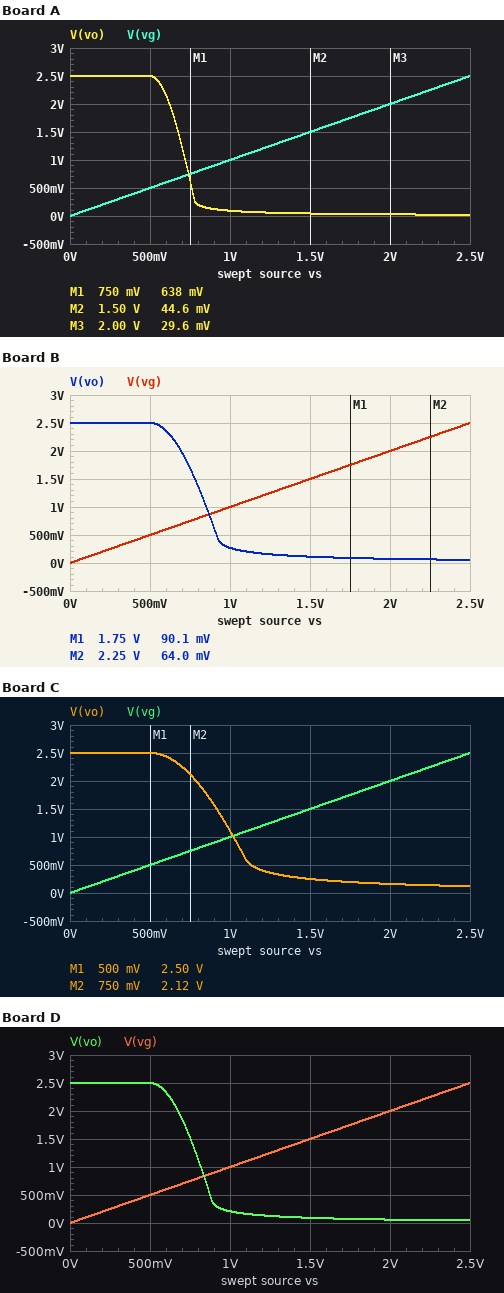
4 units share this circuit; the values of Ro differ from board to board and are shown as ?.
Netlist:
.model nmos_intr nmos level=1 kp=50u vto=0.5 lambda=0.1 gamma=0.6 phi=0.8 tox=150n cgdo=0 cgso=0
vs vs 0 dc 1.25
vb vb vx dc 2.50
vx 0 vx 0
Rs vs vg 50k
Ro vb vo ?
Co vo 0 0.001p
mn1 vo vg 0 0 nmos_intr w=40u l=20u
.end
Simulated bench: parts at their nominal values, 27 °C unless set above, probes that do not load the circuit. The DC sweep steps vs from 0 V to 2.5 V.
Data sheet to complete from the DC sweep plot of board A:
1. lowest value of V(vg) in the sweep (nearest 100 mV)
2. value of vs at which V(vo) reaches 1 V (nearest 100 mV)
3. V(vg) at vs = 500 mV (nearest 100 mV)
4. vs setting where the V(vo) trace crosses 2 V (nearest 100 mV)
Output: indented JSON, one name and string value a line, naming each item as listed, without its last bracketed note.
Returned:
{
  "lowest value of V(vg) in the sweep": "0 V",
  "value of vs at which V(vo) reaches 1 V": "700 mV",
  "V(vg) at vs = 500 mV": "500 mV",
  "vs setting where the V(vo) trace crosses 2 V": "600 mV"
}
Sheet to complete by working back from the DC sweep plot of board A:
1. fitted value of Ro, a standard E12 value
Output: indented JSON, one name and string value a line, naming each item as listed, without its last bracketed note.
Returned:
{
  "fitted value of Ro, a standard E12 value": "560 kΩ"
}
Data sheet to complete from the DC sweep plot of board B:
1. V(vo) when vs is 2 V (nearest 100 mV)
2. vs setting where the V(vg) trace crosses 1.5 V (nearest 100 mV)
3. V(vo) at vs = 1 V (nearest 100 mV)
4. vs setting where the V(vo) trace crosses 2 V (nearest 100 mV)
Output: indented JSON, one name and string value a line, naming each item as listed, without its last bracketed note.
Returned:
{
  "V(vo) when vs is 2 V": "100 mV",
  "vs setting where the V(vg) trace crosses 1.5 V": "1.5 V",
  "V(vo) at vs = 1 V": "300 mV",
  "vs setting where the V(vo) trace crosses 2 V": "700 mV"
}
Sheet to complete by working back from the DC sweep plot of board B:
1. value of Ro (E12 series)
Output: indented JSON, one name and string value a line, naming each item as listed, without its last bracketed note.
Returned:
{
  "value of Ro": "220 kΩ"
}
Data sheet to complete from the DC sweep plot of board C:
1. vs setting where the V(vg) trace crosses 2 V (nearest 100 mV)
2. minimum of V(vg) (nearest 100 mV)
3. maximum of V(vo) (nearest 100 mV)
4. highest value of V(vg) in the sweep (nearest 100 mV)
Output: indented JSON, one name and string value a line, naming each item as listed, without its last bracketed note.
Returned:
{
  "vs setting where the V(vg) trace crosses 2 V": "2.0 V",
  "minimum of V(vg)": "0 V",
  "maximum of V(vo)": "2.5 V",
  "highest value of V(vg) in the sweep": "2.5 V"
}
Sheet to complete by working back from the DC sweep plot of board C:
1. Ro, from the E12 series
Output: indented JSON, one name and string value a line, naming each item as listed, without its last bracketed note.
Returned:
{
  "Ro, from the E12 series": "100 kΩ"
}
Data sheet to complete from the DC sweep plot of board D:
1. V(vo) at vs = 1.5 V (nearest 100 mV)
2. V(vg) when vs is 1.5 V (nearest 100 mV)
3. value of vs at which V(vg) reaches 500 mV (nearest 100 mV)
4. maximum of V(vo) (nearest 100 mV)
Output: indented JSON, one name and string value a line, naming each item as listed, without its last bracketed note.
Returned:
{
  "V(vo) at vs = 1.5 V": "100 mV",
  "V(vg) when vs is 1.5 V": "1.5 V",
  "value of vs at which V(vg) reaches 500 mV": "500 mV",
  "maximum of V(vo)": "2.5 V"
}
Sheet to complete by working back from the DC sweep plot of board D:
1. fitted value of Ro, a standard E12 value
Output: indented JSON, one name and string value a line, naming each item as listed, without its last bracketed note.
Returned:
{
  "fitted value of Ro, a standard E12 value": "270 kΩ"
}
